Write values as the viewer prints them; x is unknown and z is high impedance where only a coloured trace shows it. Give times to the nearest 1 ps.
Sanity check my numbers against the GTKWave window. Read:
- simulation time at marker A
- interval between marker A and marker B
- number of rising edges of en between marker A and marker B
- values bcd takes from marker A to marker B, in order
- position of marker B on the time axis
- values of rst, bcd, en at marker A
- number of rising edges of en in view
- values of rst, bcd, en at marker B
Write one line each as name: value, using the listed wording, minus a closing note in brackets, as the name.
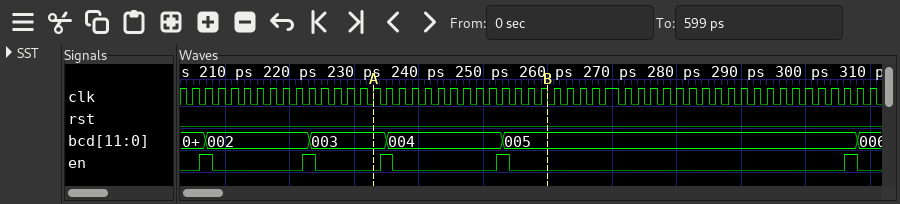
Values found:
simulation time at marker A: 233 ps
interval between marker A and marker B: 27 ps
number of rising edges of en between marker A and marker B: 2
values bcd takes from marker A to marker B, in order: 003, 004, 005
position of marker B on the time axis: 260 ps
values of rst, bcd, en at marker A: rst=0, bcd=003, en=0
number of rising edges of en in view: 5
values of rst, bcd, en at marker B: rst=0, bcd=005, en=0
